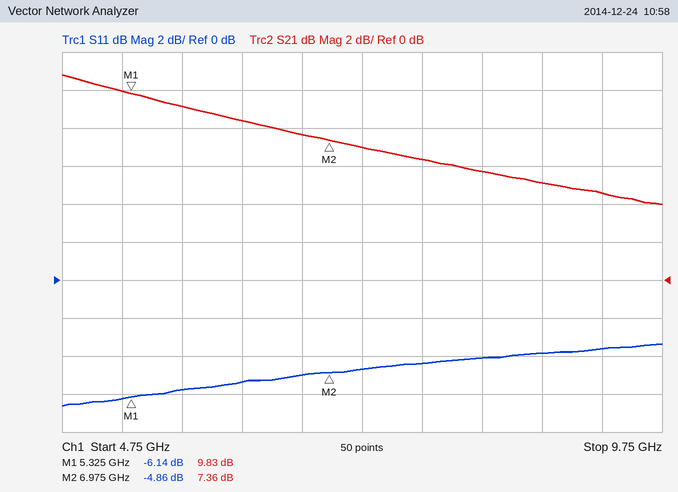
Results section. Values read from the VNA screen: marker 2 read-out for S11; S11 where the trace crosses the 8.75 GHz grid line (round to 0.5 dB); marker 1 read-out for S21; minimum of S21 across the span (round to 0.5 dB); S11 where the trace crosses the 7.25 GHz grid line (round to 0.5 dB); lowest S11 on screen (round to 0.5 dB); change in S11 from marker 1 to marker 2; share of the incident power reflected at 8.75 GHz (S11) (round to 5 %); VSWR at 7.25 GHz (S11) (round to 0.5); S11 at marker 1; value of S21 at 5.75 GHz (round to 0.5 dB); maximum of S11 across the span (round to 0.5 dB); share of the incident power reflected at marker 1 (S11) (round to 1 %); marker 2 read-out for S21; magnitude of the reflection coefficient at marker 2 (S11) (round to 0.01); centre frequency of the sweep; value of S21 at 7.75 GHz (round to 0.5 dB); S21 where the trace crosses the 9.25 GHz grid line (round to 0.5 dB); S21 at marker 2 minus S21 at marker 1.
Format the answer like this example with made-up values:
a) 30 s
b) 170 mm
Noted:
a) -4.86 dB
b) -4.0 dB
c) 9.83 dB
d) 4.0 dB
e) -4.5 dB
f) -6.5 dB
g) 1.28 dB
h) 40 %
i) 4.0
j) -6.14 dB
k) 9.0 dB
l) -3.5 dB
m) 24 %
n) 7.36 dB
o) 0.57
p) 7.25 GHz
q) 6.5 dB
r) 4.5 dB
s) -2.47 dB
